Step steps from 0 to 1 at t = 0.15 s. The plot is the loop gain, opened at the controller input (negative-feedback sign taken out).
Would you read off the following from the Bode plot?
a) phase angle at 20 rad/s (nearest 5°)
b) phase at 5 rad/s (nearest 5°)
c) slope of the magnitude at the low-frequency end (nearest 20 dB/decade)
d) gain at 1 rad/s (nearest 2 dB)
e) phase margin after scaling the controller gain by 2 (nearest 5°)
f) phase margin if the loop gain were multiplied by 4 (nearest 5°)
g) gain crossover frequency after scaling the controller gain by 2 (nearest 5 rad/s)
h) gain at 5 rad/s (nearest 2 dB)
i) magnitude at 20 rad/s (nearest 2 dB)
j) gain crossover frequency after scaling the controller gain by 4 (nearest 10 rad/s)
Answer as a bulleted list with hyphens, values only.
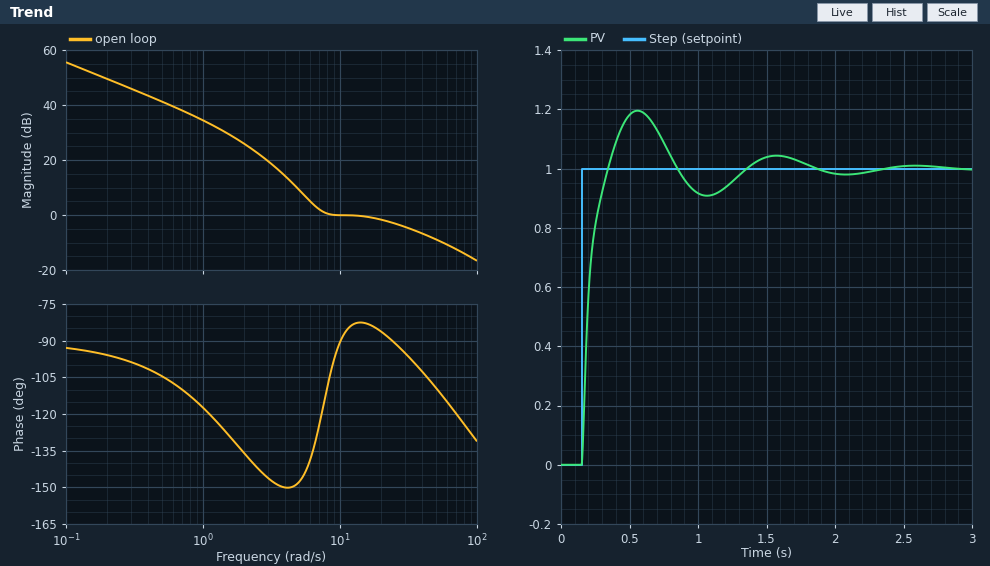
- -85°
- -150°
- -20 dB/decade
- 34 dB
- 80°
- 60°
- 35 rad/s
- 10 dB
- -2 dB
- 70 rad/s
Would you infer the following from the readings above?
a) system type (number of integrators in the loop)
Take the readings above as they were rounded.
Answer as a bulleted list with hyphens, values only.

- 1
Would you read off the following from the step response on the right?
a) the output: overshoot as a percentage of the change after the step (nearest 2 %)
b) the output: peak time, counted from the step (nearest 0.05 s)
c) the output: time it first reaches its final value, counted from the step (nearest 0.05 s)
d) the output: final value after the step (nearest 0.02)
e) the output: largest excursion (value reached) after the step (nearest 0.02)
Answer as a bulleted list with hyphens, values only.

- 20 %
- 0.40 s
- 0.20 s
- 1.00
- 1.20
